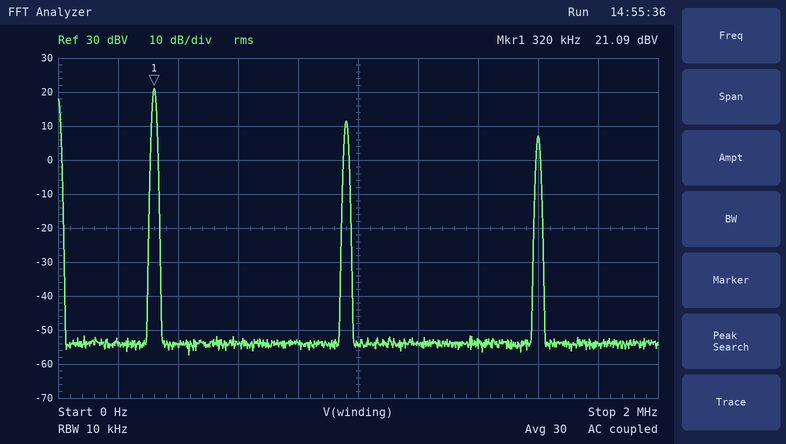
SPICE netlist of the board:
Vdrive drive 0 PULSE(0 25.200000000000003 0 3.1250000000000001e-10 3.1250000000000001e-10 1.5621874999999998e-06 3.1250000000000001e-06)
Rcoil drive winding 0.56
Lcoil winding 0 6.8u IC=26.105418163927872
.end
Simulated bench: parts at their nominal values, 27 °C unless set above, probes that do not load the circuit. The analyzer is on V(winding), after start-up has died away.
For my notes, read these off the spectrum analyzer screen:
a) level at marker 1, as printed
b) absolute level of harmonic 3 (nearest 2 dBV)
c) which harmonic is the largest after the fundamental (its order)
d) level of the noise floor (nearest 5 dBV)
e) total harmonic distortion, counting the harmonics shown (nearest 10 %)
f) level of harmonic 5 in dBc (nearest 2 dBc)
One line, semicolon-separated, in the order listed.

21.09 dBV; 12 dBV; 3; -55 dBV; 40 %; -14 dBc
